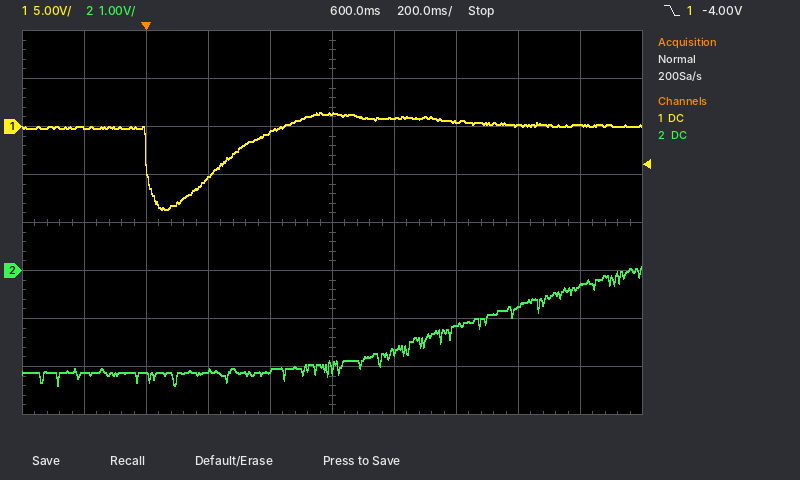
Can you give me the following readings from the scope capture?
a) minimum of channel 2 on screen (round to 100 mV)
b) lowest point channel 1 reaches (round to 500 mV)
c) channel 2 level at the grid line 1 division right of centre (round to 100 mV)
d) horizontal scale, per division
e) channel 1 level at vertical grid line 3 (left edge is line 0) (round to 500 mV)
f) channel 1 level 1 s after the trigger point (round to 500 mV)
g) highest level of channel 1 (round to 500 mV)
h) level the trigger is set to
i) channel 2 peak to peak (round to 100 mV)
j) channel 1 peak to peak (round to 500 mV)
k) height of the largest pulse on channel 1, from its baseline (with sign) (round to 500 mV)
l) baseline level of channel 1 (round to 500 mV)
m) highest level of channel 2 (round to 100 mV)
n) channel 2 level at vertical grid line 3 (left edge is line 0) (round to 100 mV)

-2.4 V
-8.5 V
-1.7 V
200 ms
-5.5 V
500 mV
1.5 V
-4.00 V
2.5 V
10.0 V
-8.5 V
0.0 V
100 mV
-2.1 V
